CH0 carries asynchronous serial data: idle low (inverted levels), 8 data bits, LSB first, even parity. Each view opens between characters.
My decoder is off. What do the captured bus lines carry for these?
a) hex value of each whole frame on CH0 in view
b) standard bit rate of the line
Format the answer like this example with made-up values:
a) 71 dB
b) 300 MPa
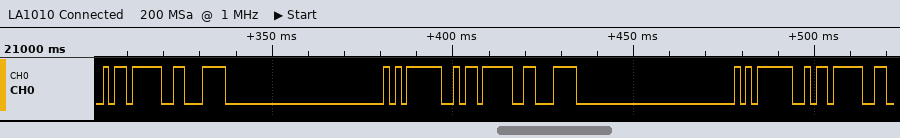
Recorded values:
a) 09, 0E, 05, 09, 0E, 05, 09
b) 600 baud
